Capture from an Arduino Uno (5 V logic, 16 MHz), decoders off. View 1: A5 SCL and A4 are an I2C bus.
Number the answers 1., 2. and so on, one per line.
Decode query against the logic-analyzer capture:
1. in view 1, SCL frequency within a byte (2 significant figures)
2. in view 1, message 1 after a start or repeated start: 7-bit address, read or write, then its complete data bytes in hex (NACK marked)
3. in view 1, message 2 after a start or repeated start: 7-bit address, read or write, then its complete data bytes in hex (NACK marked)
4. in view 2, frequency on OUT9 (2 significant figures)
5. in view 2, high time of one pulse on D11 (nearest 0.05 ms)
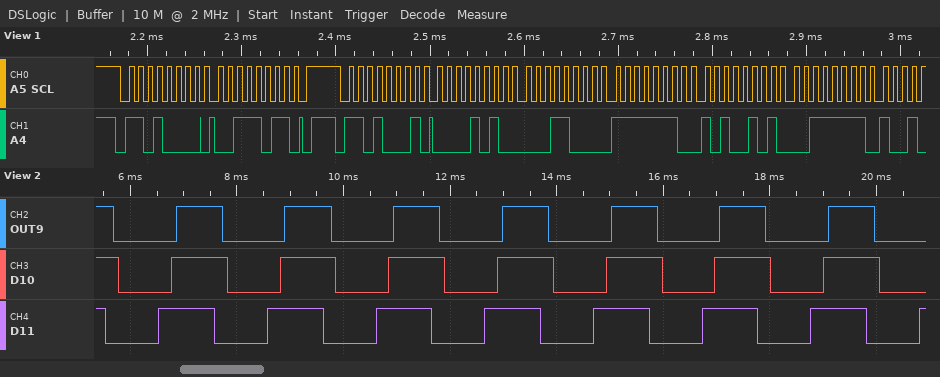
1. 100 kHz
2. 0x68 write: 3B
3. 0x68 read: 0A 18 FE A5 3F
4. 490 Hz
5. 1.05 ms
